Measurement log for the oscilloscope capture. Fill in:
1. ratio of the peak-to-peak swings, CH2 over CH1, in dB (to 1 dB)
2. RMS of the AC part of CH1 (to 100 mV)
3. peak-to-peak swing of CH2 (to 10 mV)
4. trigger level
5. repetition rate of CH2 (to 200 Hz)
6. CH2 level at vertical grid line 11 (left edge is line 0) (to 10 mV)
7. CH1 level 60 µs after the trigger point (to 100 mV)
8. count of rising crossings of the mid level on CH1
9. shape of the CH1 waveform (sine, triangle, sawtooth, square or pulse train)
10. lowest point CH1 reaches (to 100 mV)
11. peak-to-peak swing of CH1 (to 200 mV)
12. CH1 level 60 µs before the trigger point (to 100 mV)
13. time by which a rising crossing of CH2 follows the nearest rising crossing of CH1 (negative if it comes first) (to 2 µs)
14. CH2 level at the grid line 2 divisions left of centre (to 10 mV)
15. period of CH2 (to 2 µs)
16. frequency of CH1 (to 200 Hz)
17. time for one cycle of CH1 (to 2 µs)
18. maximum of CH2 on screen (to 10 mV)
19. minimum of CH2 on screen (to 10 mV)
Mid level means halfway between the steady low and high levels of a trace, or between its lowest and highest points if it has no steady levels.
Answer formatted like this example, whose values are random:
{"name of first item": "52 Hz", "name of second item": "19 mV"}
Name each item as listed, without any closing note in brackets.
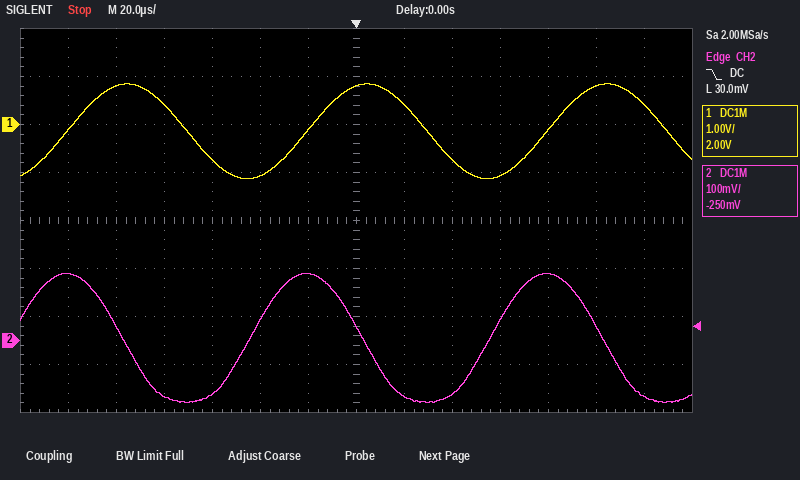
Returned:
{"ratio of the peak-to-peak swings, CH2 over CH1, in dB": "-17 dB", "RMS of the AC part of CH1": "700 mV", "peak-to-peak swing of CH2": "270 mV", "trigger level": "30.0 mV", "repetition rate of CH2": "10.0 kHz", "CH2 level at vertical grid line 11 (left edge is line 0)": "140 mV", "CH1 level 60 µs after the trigger point": "-1.1 V", "count of rising crossings of the mid level on CH1": "3", "shape of the CH1 waveform": "sine", "lowest point CH1 reaches": "-1.1 V", "peak-to-peak swing of CH1": "2.0 V", "CH1 level 60 µs before the trigger point": "-700 mV", "time by which a rising crossing of CH2 follows the nearest rising crossing of CH1 (negative if it comes first)": "-24 µs", "CH2 level at the grid line 2 divisions left of centre": "40 mV", "period of CH2": "100 µs", "frequency of CH1": "10.0 kHz", "time for one cycle of CH1": "100 µs", "maximum of CH2 on screen": "140 mV", "minimum of CH2 on screen": "-130 mV"}
